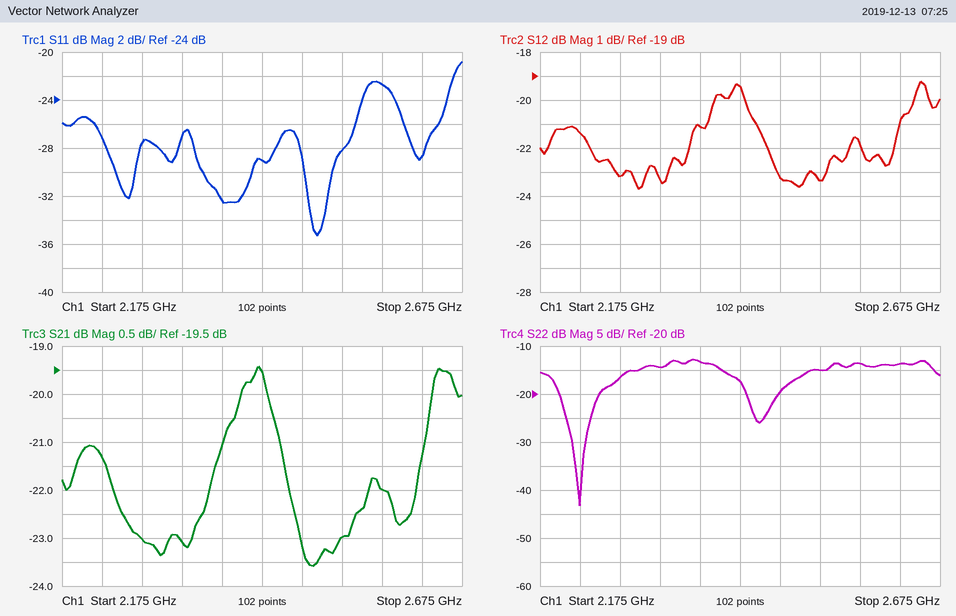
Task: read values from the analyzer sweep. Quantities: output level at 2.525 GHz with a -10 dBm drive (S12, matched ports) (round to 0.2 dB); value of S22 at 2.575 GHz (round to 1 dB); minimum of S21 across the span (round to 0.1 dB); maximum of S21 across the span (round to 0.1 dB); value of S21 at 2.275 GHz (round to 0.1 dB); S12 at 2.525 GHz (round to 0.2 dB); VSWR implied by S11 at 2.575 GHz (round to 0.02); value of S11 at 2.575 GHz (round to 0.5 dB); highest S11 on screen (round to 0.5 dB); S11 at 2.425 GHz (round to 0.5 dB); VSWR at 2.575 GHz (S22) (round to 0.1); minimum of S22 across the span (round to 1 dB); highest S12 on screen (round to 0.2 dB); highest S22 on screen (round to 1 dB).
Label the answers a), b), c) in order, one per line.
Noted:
a) -33.4 dBm
b) -14 dB
c) -23.6 dB
d) -19.4 dB
e) -23.0 dB
f) -23.4 dB
g) 1.16
h) -22.5 dB
i) -21.0 dB
j) -29.0 dB
k) 1.5
l) -43 dB
m) -19.2 dB
n) -13 dB
